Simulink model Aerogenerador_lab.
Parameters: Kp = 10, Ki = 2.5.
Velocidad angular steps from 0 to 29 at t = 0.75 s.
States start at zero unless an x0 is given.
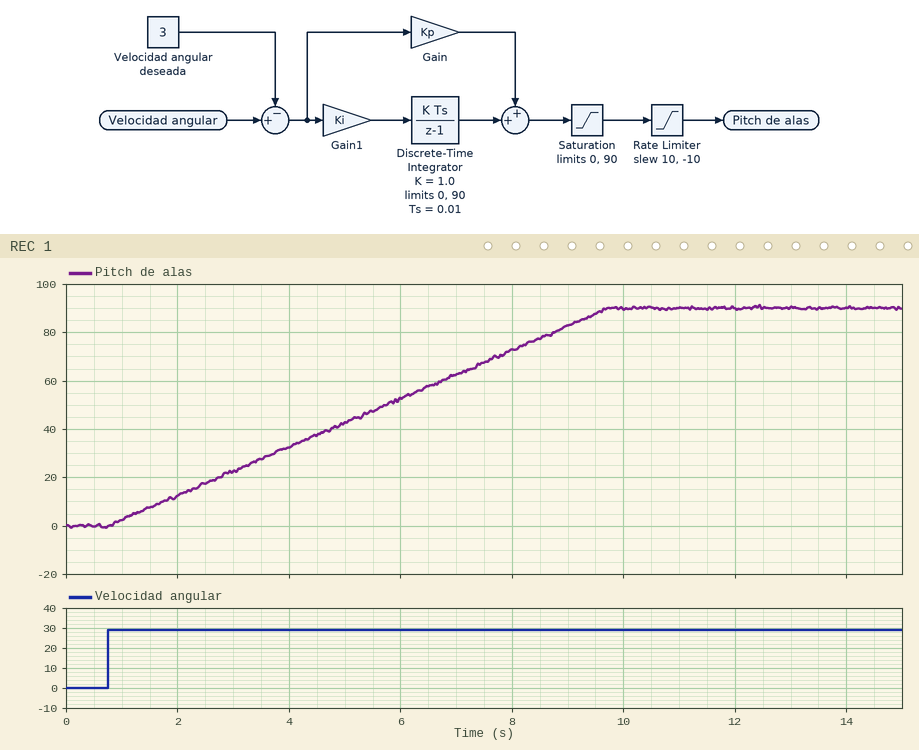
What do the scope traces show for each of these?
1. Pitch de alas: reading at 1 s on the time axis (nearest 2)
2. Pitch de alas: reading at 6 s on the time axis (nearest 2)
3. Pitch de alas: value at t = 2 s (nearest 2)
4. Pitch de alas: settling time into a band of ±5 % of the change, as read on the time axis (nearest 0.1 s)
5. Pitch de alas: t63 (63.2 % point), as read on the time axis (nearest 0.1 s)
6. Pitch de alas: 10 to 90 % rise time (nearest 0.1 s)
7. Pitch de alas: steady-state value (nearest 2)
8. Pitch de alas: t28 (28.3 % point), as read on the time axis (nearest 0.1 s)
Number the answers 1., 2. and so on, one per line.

1. 2
2. 52
3. 12
4. 9.3 s
5. 6.4 s
6. 7.2 s
7. 90
8. 3.3 s
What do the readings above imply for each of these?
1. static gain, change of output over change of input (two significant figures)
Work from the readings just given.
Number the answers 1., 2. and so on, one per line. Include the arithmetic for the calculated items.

1. (90 - 0) / (29 - 0) = 3.1
